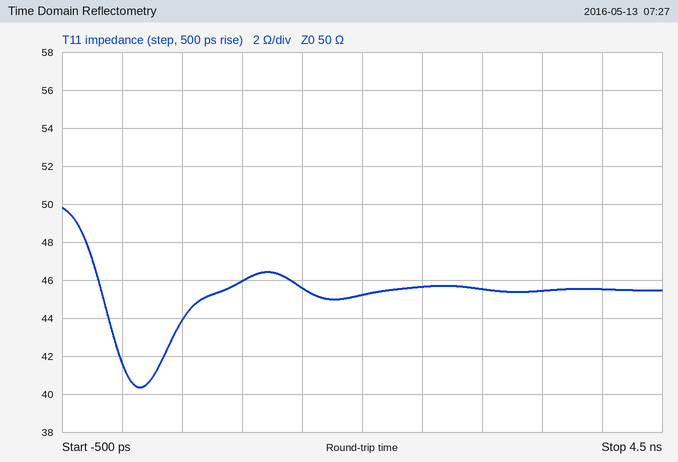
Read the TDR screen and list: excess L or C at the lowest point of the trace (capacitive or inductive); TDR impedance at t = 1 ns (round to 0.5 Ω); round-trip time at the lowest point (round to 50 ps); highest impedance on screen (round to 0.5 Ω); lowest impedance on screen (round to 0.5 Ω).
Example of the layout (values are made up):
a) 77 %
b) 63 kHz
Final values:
a) capacitive
b) 46.0 Ω
c) 150 ps
d) 50.0 Ω
e) 40.5 Ω
